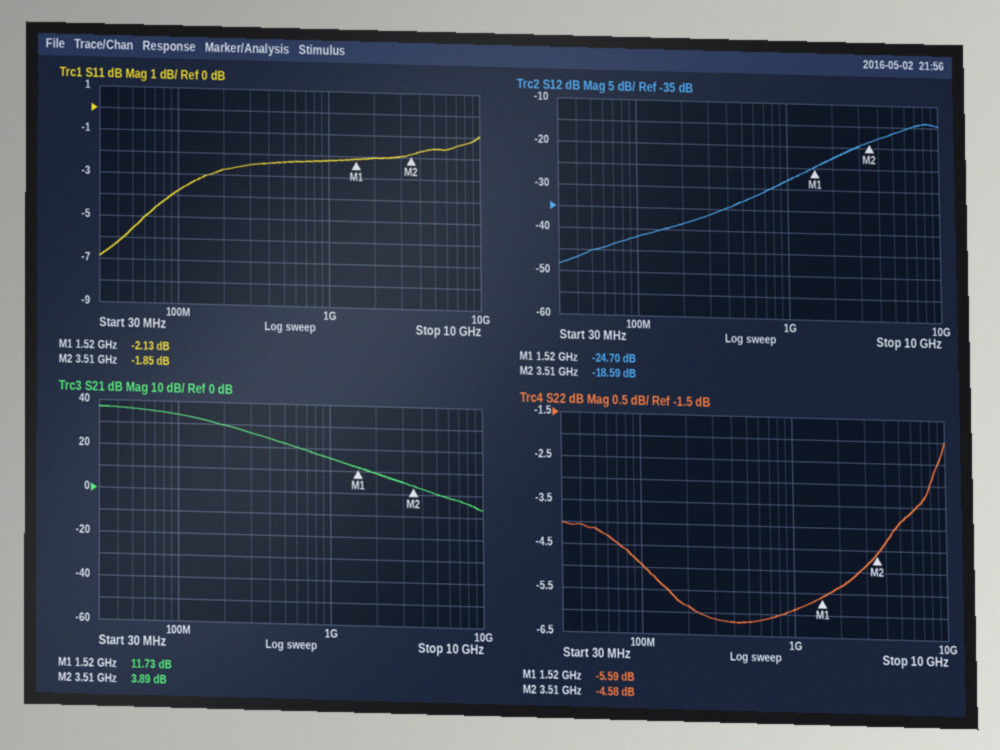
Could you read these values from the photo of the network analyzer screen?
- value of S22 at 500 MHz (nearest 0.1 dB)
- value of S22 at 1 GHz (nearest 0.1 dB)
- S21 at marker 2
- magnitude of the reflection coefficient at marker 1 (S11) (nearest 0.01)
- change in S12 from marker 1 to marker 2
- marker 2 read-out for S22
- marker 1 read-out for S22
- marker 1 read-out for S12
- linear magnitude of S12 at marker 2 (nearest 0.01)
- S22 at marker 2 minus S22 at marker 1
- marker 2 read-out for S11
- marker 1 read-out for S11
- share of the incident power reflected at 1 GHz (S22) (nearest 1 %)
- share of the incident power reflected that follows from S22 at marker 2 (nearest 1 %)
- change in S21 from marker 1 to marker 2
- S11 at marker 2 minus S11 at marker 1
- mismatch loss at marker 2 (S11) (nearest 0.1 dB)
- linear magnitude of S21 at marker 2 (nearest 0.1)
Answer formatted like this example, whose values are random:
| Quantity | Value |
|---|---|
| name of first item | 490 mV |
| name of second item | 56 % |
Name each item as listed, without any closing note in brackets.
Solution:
| Quantity | Value |
|---|---|
| value of S22 at 500 MHz | -6.2 dB |
| value of S22 at 1 GHz | -5.9 dB |
| S21 at marker 2 | 3.89 dB |
| magnitude of the reflection coefficient at marker 1 (S11) | 0.78 |
| change in S12 from marker 1 to marker 2 | 6.11 dB |
| marker 2 read-out for S22 | -4.58 dB |
| marker 1 read-out for S22 | -5.59 dB |
| marker 1 read-out for S12 | -24.70 dB |
| linear magnitude of S12 at marker 2 | 0.12 |
| S22 at marker 2 minus S22 at marker 1 | 1.01 dB |
| marker 2 read-out for S11 | -1.85 dB |
| marker 1 read-out for S11 | -2.13 dB |
| share of the incident power reflected at 1 GHz (S22) | 26 % |
| share of the incident power reflected that follows from S22 at marker 2 | 35 % |
| change in S21 from marker 1 to marker 2 | -7.84 dB |
| S11 at marker 2 minus S11 at marker 1 | 0.28 dB |
| mismatch loss at marker 2 (S11) | 4.6 dB |
| linear magnitude of S21 at marker 2 | 1.6 |
